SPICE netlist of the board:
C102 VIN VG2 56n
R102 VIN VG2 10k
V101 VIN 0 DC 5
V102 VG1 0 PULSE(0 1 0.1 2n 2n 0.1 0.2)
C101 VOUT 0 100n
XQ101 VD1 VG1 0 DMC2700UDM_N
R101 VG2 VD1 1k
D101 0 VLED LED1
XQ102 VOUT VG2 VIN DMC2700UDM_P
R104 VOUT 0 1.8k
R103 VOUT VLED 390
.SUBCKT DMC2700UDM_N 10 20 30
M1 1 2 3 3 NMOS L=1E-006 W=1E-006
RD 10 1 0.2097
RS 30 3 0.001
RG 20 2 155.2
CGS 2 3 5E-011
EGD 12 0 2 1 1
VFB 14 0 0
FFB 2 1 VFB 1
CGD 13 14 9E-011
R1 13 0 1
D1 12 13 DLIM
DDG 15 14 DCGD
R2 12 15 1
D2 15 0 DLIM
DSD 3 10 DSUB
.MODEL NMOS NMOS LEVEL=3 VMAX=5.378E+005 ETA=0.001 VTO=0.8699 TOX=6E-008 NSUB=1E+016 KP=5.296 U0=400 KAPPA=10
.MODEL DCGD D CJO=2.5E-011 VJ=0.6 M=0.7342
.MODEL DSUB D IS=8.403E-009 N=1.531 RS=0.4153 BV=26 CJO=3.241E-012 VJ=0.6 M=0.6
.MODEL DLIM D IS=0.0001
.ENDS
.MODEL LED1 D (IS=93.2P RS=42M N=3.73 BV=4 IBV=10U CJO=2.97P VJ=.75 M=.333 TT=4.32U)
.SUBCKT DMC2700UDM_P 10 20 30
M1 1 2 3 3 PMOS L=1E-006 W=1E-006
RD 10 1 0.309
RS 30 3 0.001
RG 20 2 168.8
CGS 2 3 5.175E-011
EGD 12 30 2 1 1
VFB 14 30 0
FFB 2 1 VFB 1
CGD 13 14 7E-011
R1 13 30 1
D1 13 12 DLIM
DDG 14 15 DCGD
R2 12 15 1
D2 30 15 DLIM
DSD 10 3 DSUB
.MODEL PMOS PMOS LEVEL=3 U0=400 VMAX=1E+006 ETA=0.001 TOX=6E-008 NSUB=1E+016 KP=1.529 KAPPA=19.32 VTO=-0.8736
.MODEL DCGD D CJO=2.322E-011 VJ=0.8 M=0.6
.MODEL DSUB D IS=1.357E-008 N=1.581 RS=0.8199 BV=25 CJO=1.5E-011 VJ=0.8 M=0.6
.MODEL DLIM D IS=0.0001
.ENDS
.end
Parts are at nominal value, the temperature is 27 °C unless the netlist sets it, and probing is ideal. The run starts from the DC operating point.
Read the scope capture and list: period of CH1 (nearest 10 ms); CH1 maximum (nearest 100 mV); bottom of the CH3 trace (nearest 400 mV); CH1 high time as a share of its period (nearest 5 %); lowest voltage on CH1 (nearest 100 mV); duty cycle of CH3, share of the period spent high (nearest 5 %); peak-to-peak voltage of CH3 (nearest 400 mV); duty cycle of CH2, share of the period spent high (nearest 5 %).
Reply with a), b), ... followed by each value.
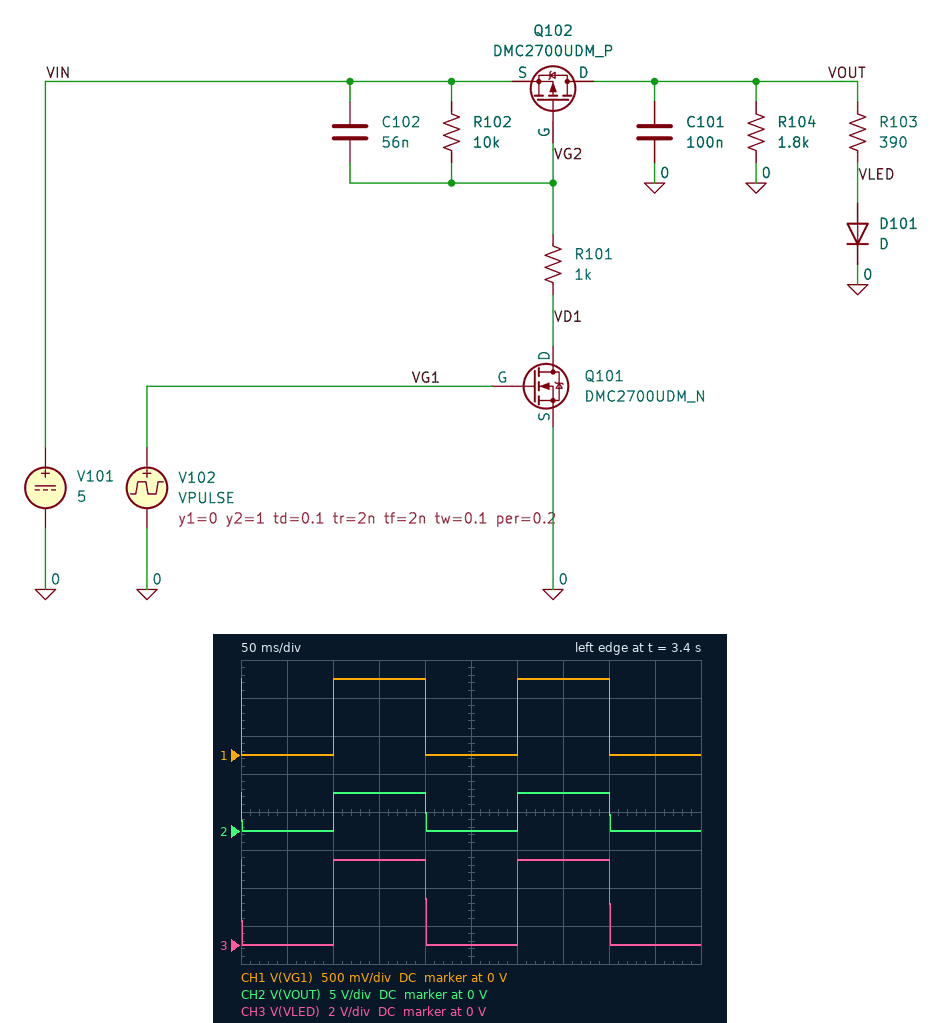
a) 200 ms
b) 1.0 V
c) 0 V
d) 50 %
e) 0 V
f) 50 %
g) 4.4 V
h) 50 %
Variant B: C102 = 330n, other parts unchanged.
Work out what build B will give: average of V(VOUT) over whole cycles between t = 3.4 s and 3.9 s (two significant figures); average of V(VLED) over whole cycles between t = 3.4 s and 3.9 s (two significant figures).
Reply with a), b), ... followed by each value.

a) 2.6 V
b) 2.4 V
